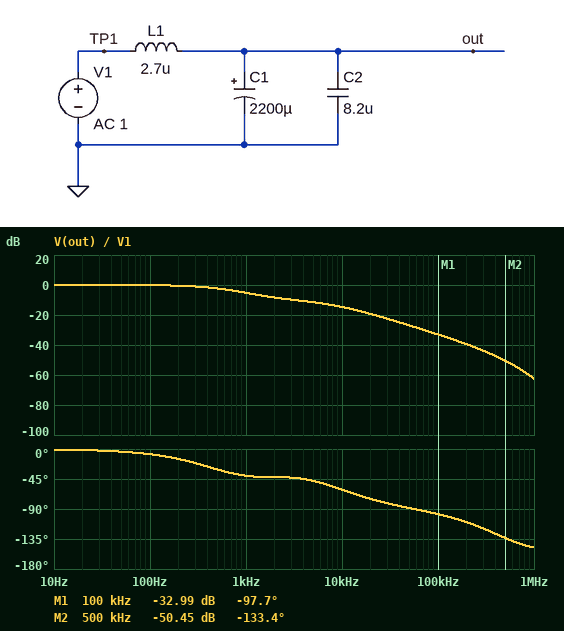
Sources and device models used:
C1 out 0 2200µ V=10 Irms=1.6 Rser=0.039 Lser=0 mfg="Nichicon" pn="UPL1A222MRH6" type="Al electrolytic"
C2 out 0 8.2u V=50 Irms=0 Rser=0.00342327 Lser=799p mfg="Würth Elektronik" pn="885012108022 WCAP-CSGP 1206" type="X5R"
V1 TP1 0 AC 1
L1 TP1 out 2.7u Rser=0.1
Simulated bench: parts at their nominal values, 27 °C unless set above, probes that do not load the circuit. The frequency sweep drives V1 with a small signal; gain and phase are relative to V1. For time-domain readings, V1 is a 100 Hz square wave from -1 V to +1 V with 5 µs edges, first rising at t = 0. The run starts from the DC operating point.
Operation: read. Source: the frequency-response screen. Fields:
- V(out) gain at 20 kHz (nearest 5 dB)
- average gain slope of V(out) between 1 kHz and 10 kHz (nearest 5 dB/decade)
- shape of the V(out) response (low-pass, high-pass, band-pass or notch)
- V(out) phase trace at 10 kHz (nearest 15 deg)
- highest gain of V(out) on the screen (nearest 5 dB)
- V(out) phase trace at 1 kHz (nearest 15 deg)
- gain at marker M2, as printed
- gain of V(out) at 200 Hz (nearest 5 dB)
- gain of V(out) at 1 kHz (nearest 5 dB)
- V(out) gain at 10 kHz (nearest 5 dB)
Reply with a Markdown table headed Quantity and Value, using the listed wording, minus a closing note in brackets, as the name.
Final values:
| Quantity | Value |
|---|---|
| V(out) gain at 20 kHz | -20 dB |
| average gain slope of V(out) between 1 kHz and 10 kHz | -10 dB/decade |
| shape of the V(out) response | low-pass |
| V(out) phase trace at 10 kHz | -60 deg |
| highest gain of V(out) on the screen | 0 dB |
| V(out) phase trace at 1 kHz | -45 deg |
| gain at marker M2, as printed | -50.45 dB |
| gain of V(out) at 200 Hz | 0 dB |
| gain of V(out) at 1 kHz | -5 dB |
| V(out) gain at 10 kHz | -15 dB |
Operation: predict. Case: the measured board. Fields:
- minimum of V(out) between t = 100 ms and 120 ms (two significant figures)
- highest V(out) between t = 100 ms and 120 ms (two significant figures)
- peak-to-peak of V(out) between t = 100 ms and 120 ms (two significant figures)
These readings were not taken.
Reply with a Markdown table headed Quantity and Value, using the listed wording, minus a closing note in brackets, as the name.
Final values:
| Quantity | Value |
|---|---|
| minimum of V(out) between t = 100 ms and 120 ms | -1.0 V |
| highest V(out) between t = 100 ms and 120 ms | 1.0 V |
| peak-to-peak of V(out) between t = 100 ms and 120 ms | 2.0 V |
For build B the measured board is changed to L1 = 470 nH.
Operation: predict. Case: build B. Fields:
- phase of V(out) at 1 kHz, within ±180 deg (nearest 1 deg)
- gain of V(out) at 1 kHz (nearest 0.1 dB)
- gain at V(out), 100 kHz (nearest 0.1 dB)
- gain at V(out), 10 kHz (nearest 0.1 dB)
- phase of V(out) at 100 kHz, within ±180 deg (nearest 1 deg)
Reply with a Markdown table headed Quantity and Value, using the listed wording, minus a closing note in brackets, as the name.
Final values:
| Quantity | Value |
|---|---|
| phase of V(out) at 1 kHz, within ±180 deg | -35 deg |
| gain of V(out) at 1 kHz | -5.5 dB |
| gain at V(out), 100 kHz | -18.5 dB |
| gain at V(out), 10 kHz | -11.0 dB |
| phase of V(out) at 100 kHz, within ±180 deg | -77 deg |
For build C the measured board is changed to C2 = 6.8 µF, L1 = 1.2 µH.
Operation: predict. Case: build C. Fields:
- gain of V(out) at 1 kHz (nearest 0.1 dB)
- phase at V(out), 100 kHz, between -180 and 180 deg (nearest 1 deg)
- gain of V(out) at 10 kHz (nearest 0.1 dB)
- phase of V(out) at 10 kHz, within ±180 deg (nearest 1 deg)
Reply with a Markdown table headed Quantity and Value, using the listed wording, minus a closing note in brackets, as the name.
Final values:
| Quantity | Value |
|---|---|
| gain of V(out) at 1 kHz | -5.4 dB |
| phase at V(out), 100 kHz, between -180 and 180 deg | -90 deg |
| gain of V(out) at 10 kHz | -11.8 dB |
| phase of V(out) at 10 kHz, within ±180 deg | -37 deg |
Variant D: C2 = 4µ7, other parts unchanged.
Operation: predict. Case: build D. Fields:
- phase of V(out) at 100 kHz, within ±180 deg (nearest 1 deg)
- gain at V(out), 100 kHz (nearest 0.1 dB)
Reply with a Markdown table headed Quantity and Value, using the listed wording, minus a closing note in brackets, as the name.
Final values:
| Quantity | Value |
|---|---|
| phase of V(out) at 100 kHz, within ±180 deg | -93 deg |
| gain at V(out), 100 kHz | -32.9 dB |
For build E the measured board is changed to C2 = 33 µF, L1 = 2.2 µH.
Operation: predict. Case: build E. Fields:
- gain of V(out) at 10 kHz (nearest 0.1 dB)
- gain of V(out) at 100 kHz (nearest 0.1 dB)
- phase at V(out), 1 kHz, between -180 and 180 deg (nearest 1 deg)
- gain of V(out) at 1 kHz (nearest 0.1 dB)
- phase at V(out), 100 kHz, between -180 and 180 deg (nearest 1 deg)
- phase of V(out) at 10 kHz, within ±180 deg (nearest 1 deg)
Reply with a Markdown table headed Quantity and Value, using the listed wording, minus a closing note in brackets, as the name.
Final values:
| Quantity | Value |
|---|---|
| gain of V(out) at 10 kHz | -13.7 dB |
| gain of V(out) at 100 kHz | -33.5 dB |
| phase at V(out), 1 kHz, between -180 and 180 deg | -39 deg |
| gain of V(out) at 1 kHz | -5.3 dB |
| phase at V(out), 100 kHz, between -180 and 180 deg | -123 deg |
| phase of V(out) at 10 kHz, within ±180 deg | -58 deg |
